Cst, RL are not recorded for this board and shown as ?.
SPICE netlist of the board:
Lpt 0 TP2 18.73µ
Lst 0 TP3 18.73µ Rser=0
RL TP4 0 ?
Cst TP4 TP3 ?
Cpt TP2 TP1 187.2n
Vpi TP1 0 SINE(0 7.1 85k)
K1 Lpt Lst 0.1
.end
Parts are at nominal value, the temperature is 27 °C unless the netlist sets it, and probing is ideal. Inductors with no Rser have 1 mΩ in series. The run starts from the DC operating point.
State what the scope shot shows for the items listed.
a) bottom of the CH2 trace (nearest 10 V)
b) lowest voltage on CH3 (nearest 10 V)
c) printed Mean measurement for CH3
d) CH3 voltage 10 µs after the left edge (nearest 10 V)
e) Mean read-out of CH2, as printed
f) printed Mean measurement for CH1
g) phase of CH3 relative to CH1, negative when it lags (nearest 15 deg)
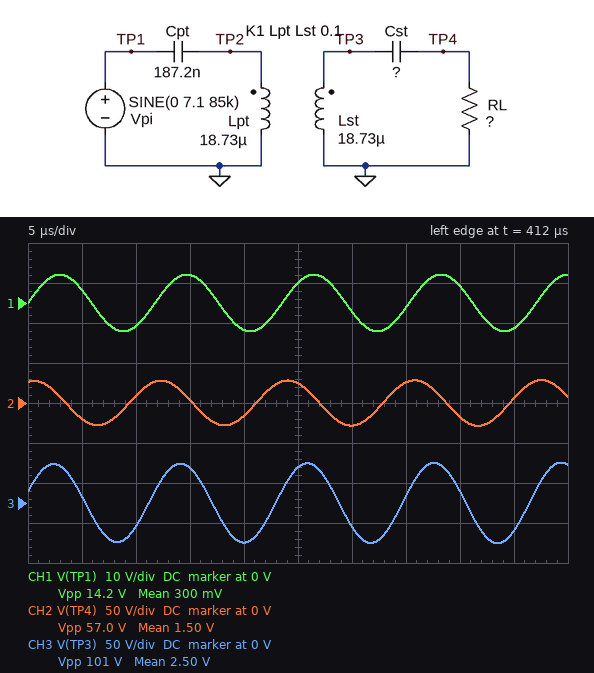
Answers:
-30 V
-50 V
2.50 V
-30 V
1.50 V
300 mV
15 deg
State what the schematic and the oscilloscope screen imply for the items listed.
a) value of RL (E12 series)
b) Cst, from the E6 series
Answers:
3.9 Ω
330 nF
